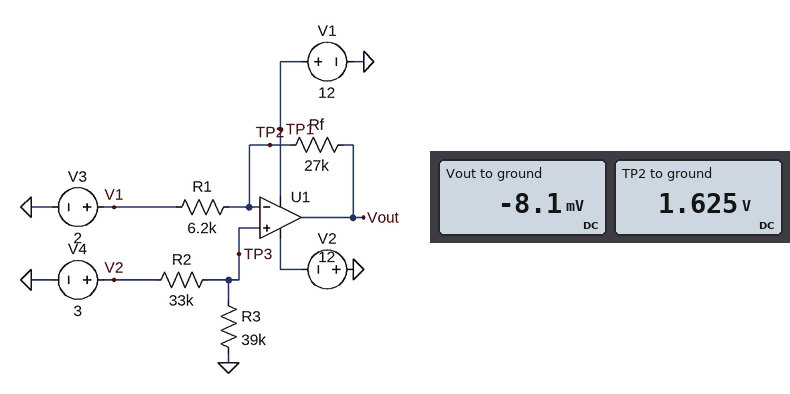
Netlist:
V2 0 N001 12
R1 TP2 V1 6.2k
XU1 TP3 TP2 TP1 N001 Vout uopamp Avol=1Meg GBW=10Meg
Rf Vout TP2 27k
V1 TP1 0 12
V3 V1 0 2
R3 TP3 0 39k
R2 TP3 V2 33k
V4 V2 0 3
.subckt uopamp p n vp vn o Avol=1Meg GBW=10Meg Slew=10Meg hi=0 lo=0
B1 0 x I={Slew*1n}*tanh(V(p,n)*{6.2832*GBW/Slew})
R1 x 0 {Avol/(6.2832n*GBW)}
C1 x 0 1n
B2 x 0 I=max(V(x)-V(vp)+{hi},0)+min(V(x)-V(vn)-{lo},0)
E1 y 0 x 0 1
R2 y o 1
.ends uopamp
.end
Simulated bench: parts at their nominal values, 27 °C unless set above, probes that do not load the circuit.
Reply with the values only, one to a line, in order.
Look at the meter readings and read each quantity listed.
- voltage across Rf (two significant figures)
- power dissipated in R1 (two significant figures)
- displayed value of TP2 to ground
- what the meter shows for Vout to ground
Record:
1.6 V
23 µW
1.625 V
-8.1 mV
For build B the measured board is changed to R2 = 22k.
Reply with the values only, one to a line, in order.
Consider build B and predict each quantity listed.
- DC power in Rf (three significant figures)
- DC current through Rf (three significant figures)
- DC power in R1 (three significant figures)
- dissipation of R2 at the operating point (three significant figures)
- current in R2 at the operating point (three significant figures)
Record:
4.72 µW
13.2 µA
1.08 µW
53.2 µW
49.2 µA
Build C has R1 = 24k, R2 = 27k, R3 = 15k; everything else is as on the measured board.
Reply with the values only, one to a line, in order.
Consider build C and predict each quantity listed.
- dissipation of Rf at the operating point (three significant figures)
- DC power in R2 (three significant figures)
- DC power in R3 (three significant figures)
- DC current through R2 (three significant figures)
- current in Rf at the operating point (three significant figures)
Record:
40.4 µW
138 µW
76.5 µW
71.4 µA
38.7 µA
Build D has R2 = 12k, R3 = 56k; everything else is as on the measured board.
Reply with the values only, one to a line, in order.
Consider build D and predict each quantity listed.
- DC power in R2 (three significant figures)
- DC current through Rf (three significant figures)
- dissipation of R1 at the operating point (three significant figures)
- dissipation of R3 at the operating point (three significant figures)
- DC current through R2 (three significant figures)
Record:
23.4 µW
75.9 µA
35.7 µW
109 µW
44.1 µA
